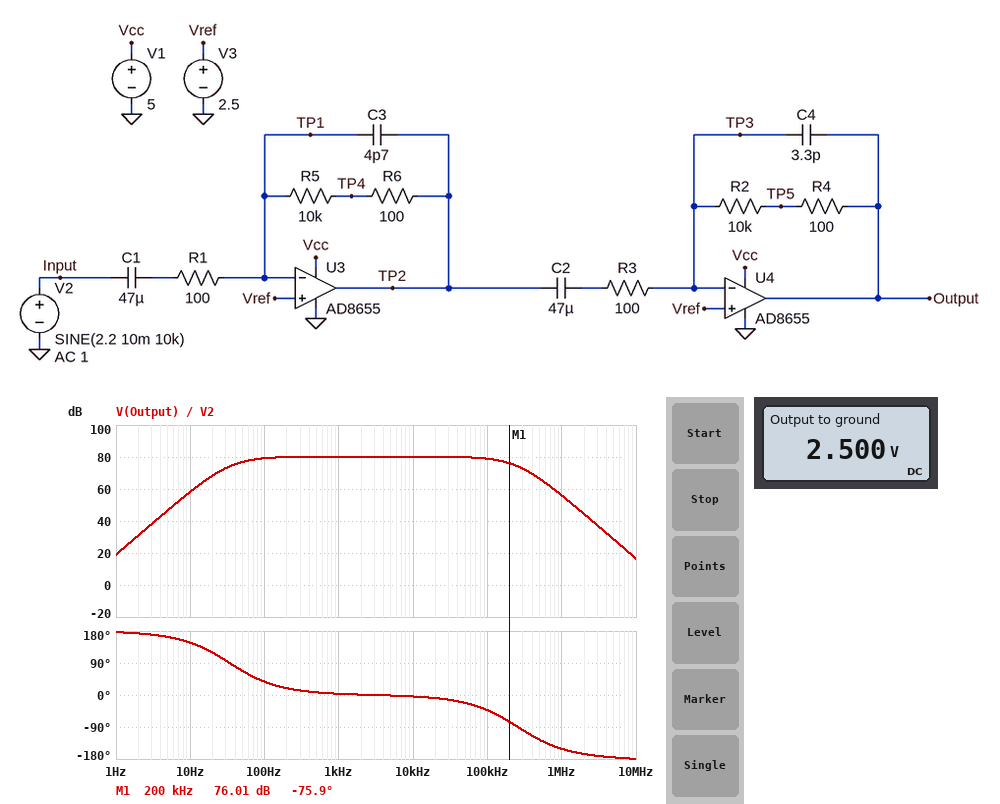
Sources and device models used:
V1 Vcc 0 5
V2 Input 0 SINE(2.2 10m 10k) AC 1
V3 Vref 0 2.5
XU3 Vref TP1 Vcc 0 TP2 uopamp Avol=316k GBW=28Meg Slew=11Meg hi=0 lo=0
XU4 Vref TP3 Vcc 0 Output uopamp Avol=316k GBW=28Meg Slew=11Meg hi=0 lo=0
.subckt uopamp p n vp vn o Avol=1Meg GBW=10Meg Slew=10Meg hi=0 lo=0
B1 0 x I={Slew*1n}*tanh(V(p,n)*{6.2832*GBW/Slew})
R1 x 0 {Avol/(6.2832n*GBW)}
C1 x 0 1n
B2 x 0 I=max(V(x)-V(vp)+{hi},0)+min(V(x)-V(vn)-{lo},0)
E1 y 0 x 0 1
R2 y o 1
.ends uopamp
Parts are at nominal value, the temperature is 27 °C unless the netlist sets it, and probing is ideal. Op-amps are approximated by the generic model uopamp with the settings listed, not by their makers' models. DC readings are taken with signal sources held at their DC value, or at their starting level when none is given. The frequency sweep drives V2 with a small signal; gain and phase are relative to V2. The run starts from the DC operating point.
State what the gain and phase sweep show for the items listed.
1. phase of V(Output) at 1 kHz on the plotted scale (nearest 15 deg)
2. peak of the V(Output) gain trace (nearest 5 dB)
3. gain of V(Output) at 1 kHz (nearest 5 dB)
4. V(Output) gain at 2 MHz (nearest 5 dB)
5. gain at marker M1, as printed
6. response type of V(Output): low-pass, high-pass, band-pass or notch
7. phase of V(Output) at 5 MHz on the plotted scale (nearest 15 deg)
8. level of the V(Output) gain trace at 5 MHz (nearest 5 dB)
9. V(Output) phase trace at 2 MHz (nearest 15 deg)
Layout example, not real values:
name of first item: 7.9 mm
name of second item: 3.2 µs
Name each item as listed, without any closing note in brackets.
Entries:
phase of V(Output) at 1 kHz on the plotted scale: 0 deg
peak of the V(Output) gain trace: 80 dB
gain of V(Output) at 1 kHz: 80 dB
V(Output) gain at 2 MHz: 45 dB
gain at marker M1, as printed: 76.01 dB
response type of V(Output): low-pass, high-pass, band-pass or notch: band-pass
phase of V(Output) at 5 MHz on the plotted scale: -180 deg
level of the V(Output) gain trace at 5 MHz: 30 dB
V(Output) phase trace at 2 MHz: -165 deg
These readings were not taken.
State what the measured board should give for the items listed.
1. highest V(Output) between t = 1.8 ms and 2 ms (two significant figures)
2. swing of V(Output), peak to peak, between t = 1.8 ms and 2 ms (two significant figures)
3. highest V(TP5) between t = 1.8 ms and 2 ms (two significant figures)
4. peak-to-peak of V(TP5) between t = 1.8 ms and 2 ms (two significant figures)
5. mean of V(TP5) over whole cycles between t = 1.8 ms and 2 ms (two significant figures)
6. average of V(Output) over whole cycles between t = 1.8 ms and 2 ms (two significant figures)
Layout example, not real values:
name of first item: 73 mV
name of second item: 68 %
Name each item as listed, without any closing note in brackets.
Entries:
highest V(Output) between t = 1.8 ms and 2 ms: 5.0 V
swing of V(Output), peak to peak, between t = 1.8 ms and 2 ms: 5.0 V
highest V(TP5) between t = 1.8 ms and 2 ms: 5.0 V
peak-to-peak of V(TP5) between t = 1.8 ms and 2 ms: 5.0 V
mean of V(TP5) over whole cycles between t = 1.8 ms and 2 ms: 2.5 V
average of V(Output) over whole cycles between t = 1.8 ms and 2 ms: 2.5 V
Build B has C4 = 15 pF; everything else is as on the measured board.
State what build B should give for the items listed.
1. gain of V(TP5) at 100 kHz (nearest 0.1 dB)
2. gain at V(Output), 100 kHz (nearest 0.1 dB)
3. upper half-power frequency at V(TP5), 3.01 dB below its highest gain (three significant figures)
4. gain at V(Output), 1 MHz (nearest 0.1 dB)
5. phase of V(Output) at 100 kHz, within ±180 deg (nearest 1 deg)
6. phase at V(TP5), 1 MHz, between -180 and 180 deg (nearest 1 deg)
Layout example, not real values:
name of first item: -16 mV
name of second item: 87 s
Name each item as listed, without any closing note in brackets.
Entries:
gain of V(TP5) at 100 kHz: 78.6 dB
gain at V(Output), 100 kHz: 78.7 dB
upper half-power frequency at V(TP5), 3.01 dB below its highest gain: 150 kHz
gain at V(Output), 1 MHz: 54.5 dB
phase of V(Output) at 100 kHz, within ±180 deg: -46 deg
phase at V(TP5), 1 MHz, between -180 and 180 deg: -154 deg
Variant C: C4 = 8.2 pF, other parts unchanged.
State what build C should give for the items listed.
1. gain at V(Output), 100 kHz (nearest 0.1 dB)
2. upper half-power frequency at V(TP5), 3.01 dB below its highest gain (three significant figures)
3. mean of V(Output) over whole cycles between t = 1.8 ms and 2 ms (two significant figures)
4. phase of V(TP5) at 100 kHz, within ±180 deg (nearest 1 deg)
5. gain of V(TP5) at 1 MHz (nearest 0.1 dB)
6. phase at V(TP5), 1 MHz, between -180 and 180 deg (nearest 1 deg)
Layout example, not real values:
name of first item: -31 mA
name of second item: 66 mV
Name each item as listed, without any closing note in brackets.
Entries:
gain at V(Output), 100 kHz: 78.8 dB
upper half-power frequency at V(TP5), 3.01 dB below its highest gain: 158 kHz
mean of V(Output) over whole cycles between t = 1.8 ms and 2 ms: 2.5 V
phase of V(TP5) at 100 kHz, within ±180 deg: -44 deg
gain of V(TP5) at 1 MHz: 55.3 dB
phase at V(TP5), 1 MHz, between -180 and 180 deg: -153 deg
